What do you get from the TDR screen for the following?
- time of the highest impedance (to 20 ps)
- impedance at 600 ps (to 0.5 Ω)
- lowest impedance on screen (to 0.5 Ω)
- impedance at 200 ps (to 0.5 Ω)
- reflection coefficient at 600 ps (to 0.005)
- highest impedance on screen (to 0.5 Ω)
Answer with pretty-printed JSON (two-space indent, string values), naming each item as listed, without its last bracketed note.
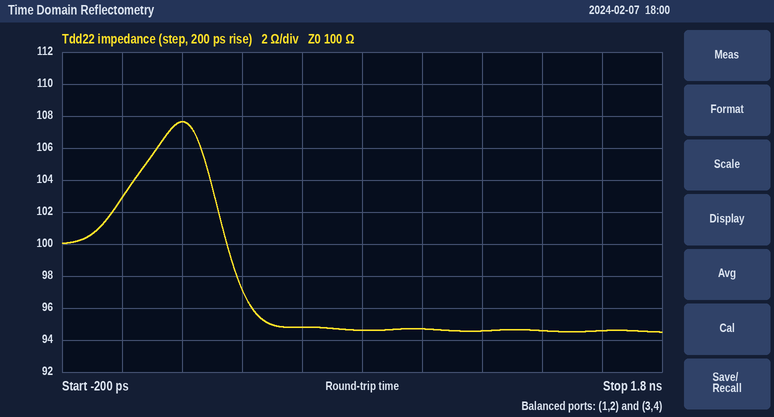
{
  "time of the highest impedance": "200 ps",
  "impedance at 600 ps": "95.0 Ω",
  "lowest impedance on screen": "94.5 Ω",
  "impedance at 200 ps": "107.5 Ω",
  "reflection coefficient at 600 ps": "-0.025",
  "highest impedance on screen": "107.5 Ω"
}
